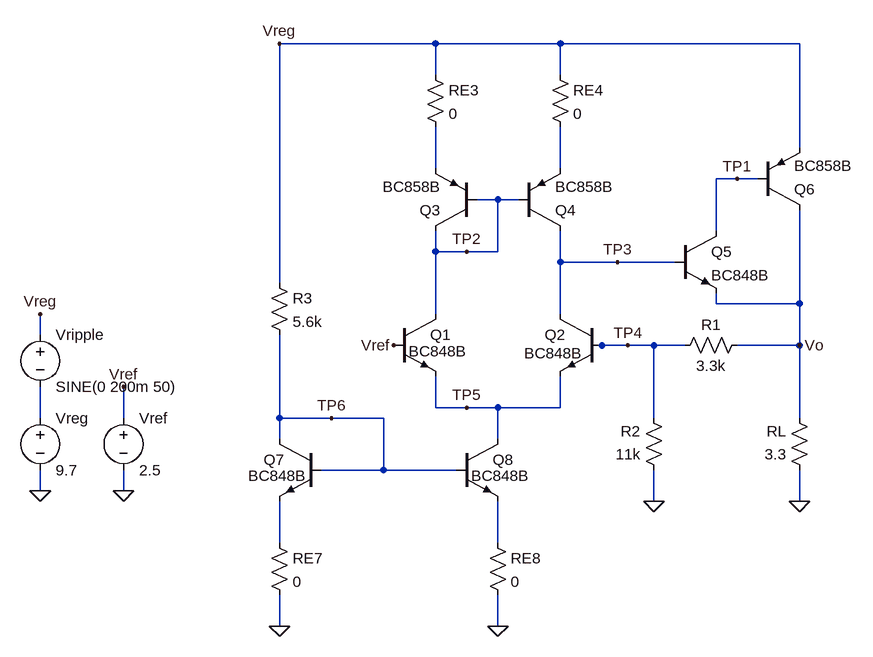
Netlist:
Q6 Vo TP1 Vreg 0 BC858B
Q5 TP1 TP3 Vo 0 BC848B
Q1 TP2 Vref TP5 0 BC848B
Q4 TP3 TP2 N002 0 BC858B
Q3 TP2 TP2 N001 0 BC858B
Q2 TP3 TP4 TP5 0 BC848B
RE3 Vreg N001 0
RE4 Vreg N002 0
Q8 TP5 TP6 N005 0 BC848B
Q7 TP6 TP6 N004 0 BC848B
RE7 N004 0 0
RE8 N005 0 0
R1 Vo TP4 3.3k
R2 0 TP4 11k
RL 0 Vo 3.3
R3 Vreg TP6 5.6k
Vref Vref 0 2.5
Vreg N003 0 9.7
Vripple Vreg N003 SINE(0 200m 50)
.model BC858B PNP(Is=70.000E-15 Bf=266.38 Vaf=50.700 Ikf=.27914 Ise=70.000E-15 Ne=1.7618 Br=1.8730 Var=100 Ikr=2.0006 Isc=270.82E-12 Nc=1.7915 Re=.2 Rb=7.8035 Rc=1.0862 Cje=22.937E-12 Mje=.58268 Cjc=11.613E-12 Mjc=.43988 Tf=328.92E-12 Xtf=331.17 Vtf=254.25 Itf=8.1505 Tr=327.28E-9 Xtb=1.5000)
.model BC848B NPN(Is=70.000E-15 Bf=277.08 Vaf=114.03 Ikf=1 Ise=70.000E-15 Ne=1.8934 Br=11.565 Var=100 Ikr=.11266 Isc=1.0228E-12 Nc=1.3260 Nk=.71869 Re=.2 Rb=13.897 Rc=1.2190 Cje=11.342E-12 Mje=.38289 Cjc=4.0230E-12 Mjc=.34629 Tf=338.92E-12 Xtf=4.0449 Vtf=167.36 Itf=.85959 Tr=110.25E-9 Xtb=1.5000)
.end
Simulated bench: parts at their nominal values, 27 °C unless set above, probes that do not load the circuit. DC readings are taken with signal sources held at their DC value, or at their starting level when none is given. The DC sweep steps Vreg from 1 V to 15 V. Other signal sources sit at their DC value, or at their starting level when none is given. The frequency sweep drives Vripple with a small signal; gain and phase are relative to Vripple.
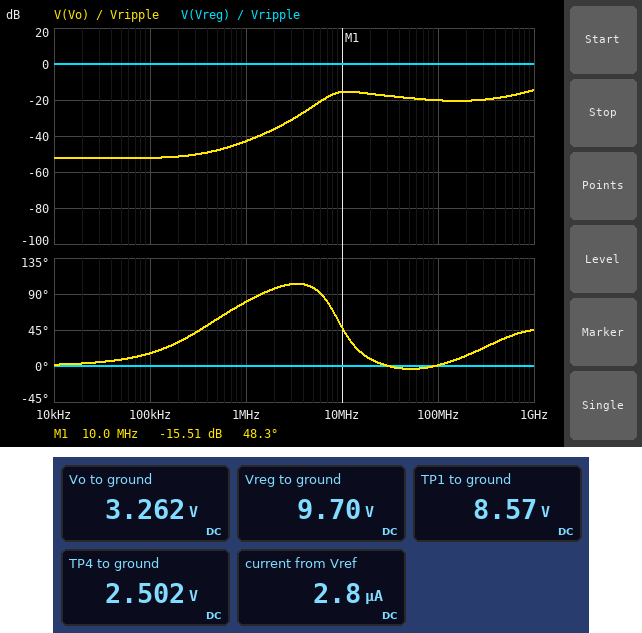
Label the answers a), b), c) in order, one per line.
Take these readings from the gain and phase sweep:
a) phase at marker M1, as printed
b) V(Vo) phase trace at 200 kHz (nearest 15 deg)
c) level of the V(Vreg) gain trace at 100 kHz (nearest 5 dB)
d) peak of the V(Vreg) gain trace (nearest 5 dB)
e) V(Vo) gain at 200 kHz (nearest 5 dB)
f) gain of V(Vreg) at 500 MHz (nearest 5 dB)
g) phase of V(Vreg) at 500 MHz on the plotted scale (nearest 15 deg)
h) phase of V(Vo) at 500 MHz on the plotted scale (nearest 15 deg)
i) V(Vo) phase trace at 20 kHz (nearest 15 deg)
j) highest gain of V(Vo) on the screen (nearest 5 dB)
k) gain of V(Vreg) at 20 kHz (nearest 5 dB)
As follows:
a) 48.3 deg
b) 30 deg
c) 0 dB
d) 0 dB
e) -50 dB
f) 0 dB
g) 0 deg
h) 30 deg
i) 0 deg
j) -15 dB
k) 0 dB
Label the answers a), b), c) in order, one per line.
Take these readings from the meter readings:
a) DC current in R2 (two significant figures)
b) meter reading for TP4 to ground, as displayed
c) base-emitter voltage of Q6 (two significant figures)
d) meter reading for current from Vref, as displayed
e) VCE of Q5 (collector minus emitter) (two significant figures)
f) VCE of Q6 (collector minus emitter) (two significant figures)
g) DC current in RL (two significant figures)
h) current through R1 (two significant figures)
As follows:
a) 230 µA
b) 2.502 V
c) -1.1 V
d) 2.8 µA
e) 5.3 V
f) -6.4 V
g) 990 mA
h) 230 µA
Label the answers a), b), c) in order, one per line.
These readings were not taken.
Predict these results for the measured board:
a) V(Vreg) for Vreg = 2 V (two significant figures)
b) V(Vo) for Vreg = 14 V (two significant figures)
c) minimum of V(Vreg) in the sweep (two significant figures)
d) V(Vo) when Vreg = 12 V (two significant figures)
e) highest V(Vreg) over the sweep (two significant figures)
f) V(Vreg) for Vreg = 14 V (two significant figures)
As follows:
a) 2.0 V
b) 3.3 V
c) 1.0 V
d) 3.3 V
e) 15 V
f) 14 V
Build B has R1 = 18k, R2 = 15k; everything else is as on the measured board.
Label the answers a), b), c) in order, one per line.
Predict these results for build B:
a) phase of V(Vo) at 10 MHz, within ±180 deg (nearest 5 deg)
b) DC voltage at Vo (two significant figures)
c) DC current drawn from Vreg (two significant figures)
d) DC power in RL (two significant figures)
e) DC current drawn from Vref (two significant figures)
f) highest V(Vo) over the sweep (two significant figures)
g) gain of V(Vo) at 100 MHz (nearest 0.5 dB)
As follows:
a) 20 deg
b) 5.5 V
c) 1.7 A
d) 9.3 W
e) 3.0 µA
f) 5.6 V
g) -17.5 dB
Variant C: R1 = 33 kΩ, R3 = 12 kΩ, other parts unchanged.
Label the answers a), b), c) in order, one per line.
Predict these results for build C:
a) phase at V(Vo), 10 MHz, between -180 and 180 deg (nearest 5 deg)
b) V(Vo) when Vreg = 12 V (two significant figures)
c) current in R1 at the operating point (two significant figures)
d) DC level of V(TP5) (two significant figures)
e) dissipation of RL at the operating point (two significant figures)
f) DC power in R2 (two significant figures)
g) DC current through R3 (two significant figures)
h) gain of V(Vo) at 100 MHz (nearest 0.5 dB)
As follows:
a) 0 deg
b) 8.7 V
c) 160 µA
d) 1.9 V
e) 15 W
f) 280 µW
g) 760 µA
h) -2.5 dB
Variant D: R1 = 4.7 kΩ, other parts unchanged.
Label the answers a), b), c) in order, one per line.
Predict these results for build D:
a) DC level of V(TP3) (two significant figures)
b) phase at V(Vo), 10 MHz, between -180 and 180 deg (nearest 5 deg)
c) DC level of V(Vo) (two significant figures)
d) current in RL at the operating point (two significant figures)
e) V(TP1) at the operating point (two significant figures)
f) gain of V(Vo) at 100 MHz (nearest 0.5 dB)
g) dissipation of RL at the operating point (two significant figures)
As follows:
a) 4.3 V
b) 35 deg
c) 3.6 V
d) 1.1 A
e) 8.5 V
f) -19.5 dB
g) 3.9 W
